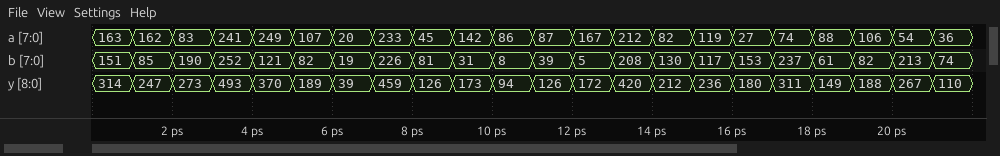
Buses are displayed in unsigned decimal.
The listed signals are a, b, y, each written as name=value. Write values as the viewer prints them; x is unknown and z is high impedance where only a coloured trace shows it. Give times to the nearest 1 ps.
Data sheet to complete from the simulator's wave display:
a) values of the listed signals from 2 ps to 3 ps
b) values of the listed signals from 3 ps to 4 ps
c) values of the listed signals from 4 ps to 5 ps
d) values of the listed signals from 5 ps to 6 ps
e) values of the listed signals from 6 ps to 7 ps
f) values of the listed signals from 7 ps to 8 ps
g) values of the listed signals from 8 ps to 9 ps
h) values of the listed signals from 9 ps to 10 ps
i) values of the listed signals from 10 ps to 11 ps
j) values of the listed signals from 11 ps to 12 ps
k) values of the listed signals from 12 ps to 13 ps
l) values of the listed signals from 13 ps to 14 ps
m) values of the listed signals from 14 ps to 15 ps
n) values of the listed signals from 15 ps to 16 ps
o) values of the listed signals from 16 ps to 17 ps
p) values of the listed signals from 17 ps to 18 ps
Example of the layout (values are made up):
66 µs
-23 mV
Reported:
a=83, b=190, y=273
a=241, b=252, y=493
a=249, b=121, y=370
a=107, b=82, y=189
a=20, b=19, y=39
a=233, b=226, y=459
a=45, b=81, y=126
a=142, b=31, y=173
a=86, b=8, y=94
a=87, b=39, y=126
a=167, b=5, y=172
a=212, b=208, y=420
a=82, b=130, y=212
a=119, b=117, y=236
a=27, b=153, y=180
a=74, b=237, y=311
